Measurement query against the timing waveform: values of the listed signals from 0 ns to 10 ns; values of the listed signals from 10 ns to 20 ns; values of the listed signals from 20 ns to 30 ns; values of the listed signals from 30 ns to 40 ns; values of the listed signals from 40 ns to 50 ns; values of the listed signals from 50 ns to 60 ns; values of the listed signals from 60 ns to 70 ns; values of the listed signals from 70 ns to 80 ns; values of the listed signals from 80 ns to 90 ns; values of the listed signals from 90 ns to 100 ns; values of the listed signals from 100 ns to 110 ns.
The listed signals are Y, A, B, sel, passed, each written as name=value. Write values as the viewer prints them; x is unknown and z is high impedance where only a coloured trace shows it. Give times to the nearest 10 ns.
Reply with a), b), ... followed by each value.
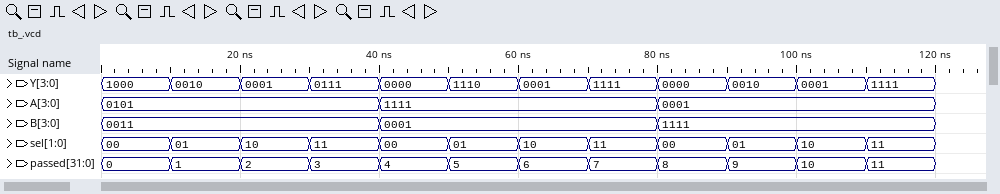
a) Y=1000, A=0101, B=0011, sel=00, passed=0
b) Y=0010, A=0101, B=0011, sel=01, passed=1
c) Y=0001, A=0101, B=0011, sel=10, passed=2
d) Y=0111, A=0101, B=0011, sel=11, passed=3
e) Y=0000, A=1111, B=0001, sel=00, passed=4
f) Y=1110, A=1111, B=0001, sel=01, passed=5
g) Y=0001, A=1111, B=0001, sel=10, passed=6
h) Y=1111, A=1111, B=0001, sel=11, passed=7
i) Y=0000, A=0001, B=1111, sel=00, passed=8
j) Y=0010, A=0001, B=1111, sel=01, passed=9
k) Y=0001, A=0001, B=1111, sel=10, passed=10
